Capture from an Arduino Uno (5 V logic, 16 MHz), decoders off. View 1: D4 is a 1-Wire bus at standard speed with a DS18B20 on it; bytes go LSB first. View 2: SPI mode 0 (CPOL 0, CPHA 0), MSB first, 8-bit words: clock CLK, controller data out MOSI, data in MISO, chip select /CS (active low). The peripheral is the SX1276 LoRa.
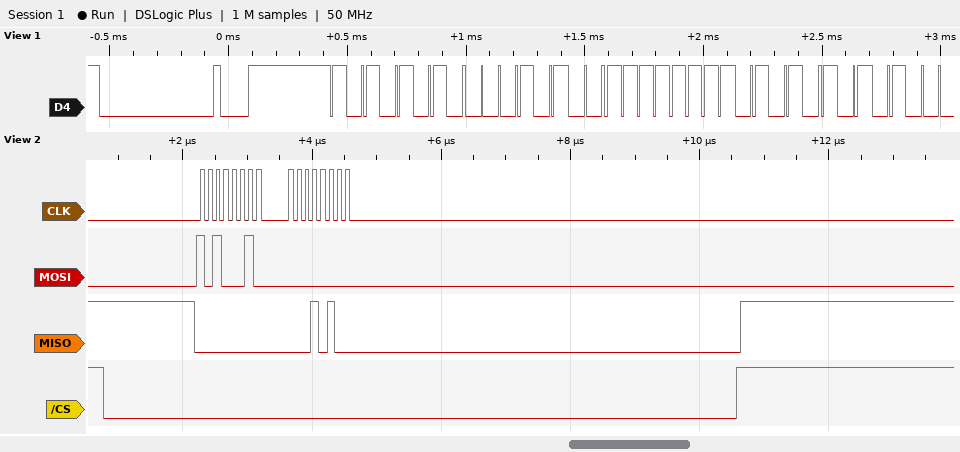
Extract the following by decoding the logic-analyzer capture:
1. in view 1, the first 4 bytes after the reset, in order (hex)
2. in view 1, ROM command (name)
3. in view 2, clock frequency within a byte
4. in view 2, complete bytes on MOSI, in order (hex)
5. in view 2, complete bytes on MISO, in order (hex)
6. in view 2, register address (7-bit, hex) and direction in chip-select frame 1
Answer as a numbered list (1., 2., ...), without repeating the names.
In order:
1. 55 28 FF AA
2. Match ROM
3. 8 MHz
4. A2 00
5. 00 14
6. 0x22 write
